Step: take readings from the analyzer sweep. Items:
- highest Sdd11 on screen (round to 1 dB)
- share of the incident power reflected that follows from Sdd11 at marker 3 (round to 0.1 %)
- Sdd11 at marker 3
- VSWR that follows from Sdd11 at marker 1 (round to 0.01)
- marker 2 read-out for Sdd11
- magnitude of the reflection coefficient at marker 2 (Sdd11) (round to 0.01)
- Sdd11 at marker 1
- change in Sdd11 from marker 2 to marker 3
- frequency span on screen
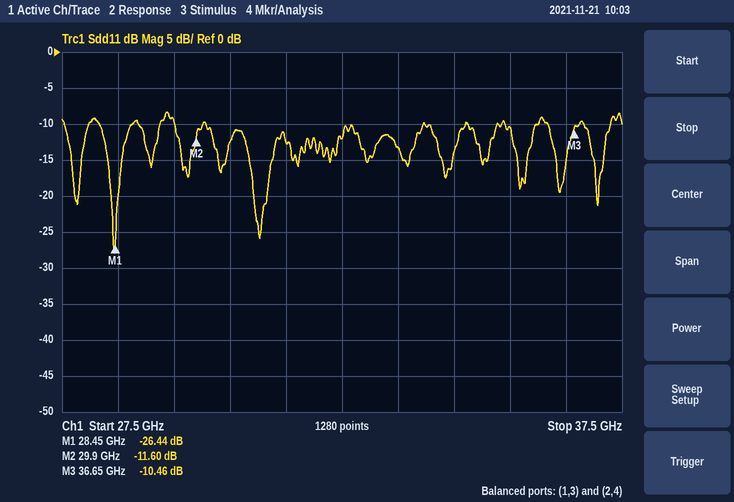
-8 dB
9.0 %
-10.46 dB
1.10
-11.60 dB
0.26
-26.44 dB
1.14 dB
10 GHz
